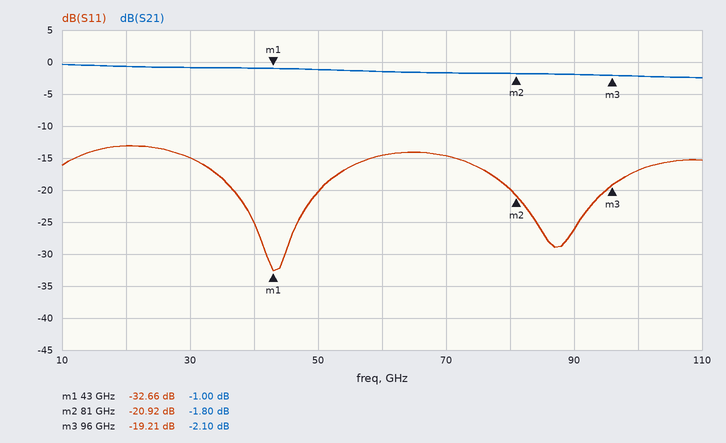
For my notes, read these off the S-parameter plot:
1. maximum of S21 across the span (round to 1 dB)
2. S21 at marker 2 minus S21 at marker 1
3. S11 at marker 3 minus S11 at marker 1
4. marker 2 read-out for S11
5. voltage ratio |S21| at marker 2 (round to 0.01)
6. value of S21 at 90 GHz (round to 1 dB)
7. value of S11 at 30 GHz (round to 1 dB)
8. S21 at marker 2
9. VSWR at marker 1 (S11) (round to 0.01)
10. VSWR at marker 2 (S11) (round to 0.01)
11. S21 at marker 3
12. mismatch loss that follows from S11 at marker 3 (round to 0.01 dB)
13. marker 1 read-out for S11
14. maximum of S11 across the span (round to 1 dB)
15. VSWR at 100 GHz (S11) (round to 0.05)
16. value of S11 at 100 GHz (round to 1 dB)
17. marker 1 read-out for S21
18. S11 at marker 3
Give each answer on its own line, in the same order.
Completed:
0 dB
-0.80 dB
13.45 dB
-20.92 dB
0.81
-2 dB
-15 dB
-1.80 dB
1.05
1.20
-2.10 dB
0.05 dB
-32.66 dB
-13 dB
1.35
-17 dB
-1.00 dB
-19.21 dB
